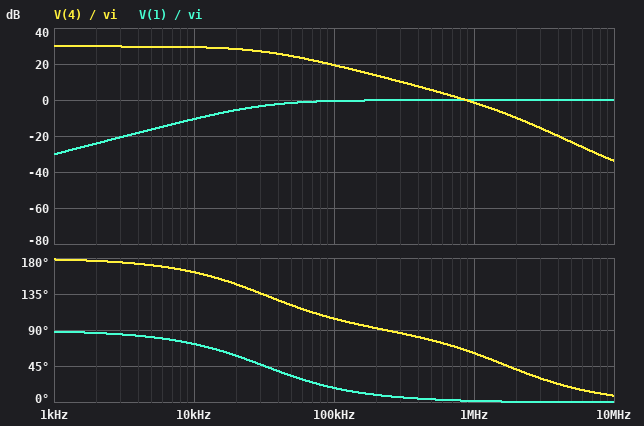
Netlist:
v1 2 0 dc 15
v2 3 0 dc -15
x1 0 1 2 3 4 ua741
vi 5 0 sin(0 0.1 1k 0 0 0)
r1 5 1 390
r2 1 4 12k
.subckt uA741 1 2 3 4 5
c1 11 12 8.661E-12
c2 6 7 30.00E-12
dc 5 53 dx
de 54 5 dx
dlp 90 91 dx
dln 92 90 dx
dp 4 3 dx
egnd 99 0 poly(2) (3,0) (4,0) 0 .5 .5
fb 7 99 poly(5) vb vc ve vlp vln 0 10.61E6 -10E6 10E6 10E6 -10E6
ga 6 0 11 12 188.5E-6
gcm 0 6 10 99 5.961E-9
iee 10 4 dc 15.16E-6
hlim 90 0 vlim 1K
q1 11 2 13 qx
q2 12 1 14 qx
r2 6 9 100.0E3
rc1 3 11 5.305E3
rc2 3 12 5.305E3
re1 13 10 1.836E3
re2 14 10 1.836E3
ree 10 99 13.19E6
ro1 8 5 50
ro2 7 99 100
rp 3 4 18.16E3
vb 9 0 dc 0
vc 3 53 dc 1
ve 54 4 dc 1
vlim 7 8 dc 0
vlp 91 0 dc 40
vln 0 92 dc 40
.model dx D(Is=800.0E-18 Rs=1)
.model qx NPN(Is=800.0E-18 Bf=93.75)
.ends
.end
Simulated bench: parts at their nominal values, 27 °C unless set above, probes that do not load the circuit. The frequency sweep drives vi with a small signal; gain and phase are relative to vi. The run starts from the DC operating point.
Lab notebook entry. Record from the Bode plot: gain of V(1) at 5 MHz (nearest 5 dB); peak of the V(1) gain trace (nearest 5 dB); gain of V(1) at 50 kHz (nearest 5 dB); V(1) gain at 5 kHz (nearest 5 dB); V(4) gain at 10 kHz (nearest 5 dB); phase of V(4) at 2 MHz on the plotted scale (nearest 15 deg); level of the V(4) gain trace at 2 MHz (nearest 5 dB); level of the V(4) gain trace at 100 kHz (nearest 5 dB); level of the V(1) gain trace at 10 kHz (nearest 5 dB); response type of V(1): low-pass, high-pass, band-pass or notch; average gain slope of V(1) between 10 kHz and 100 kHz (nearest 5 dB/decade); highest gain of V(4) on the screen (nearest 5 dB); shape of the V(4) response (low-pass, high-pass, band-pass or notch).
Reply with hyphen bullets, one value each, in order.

- 0 dB
- 0 dB
- 0 dB
- -15 dB
- 30 dB
- 45 deg
- -10 dB
- 20 dB
- -10 dB
- high-pass
- 10 dB/decade
- 30 dB
- low-pass
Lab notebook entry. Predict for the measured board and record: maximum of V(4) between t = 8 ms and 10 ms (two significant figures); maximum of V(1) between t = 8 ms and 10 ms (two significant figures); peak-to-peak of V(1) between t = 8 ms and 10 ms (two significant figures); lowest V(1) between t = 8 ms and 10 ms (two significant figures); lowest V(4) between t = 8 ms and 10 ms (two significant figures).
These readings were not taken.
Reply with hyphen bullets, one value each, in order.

- 3.1 V
- 3.1 mV
- 6.2 mV
- -3.1 mV
- -3.1 V
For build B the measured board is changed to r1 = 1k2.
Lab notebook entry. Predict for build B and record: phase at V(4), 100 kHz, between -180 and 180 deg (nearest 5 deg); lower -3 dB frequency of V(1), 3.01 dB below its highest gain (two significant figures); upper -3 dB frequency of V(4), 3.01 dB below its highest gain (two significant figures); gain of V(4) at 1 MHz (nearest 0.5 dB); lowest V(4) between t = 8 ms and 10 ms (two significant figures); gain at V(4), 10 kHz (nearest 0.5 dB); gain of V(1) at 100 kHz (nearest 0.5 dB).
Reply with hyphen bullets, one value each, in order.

- 130 deg
- 92 kHz
- 95 kHz
- -2.0 dB
- -1.0 V
- 20.0 dB
- -3.0 dB
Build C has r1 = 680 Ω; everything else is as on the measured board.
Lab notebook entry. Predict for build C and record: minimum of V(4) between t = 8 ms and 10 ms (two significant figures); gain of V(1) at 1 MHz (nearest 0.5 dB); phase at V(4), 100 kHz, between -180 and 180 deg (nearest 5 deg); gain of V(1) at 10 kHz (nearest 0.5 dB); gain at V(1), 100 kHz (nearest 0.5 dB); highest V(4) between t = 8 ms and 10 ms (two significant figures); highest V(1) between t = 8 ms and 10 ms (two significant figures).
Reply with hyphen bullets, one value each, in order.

- -1.8 V
- -0.5 dB
- 115 deg
- -15.0 dB
- -1.5 dB
- 1.8 V
- 1.8 mV
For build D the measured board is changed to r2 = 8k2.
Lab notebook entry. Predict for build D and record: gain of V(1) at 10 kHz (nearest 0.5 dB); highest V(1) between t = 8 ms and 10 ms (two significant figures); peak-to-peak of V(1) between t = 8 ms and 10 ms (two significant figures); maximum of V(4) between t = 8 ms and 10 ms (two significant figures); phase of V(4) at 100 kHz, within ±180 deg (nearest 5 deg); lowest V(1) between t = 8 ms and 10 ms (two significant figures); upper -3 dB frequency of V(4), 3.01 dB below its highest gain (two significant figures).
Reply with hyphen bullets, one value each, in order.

- -13.5 dB
- 2.1 mV
- 4.2 mV
- 2.1 V
- 110 deg
- -2.1 mV
- 46 kHz
